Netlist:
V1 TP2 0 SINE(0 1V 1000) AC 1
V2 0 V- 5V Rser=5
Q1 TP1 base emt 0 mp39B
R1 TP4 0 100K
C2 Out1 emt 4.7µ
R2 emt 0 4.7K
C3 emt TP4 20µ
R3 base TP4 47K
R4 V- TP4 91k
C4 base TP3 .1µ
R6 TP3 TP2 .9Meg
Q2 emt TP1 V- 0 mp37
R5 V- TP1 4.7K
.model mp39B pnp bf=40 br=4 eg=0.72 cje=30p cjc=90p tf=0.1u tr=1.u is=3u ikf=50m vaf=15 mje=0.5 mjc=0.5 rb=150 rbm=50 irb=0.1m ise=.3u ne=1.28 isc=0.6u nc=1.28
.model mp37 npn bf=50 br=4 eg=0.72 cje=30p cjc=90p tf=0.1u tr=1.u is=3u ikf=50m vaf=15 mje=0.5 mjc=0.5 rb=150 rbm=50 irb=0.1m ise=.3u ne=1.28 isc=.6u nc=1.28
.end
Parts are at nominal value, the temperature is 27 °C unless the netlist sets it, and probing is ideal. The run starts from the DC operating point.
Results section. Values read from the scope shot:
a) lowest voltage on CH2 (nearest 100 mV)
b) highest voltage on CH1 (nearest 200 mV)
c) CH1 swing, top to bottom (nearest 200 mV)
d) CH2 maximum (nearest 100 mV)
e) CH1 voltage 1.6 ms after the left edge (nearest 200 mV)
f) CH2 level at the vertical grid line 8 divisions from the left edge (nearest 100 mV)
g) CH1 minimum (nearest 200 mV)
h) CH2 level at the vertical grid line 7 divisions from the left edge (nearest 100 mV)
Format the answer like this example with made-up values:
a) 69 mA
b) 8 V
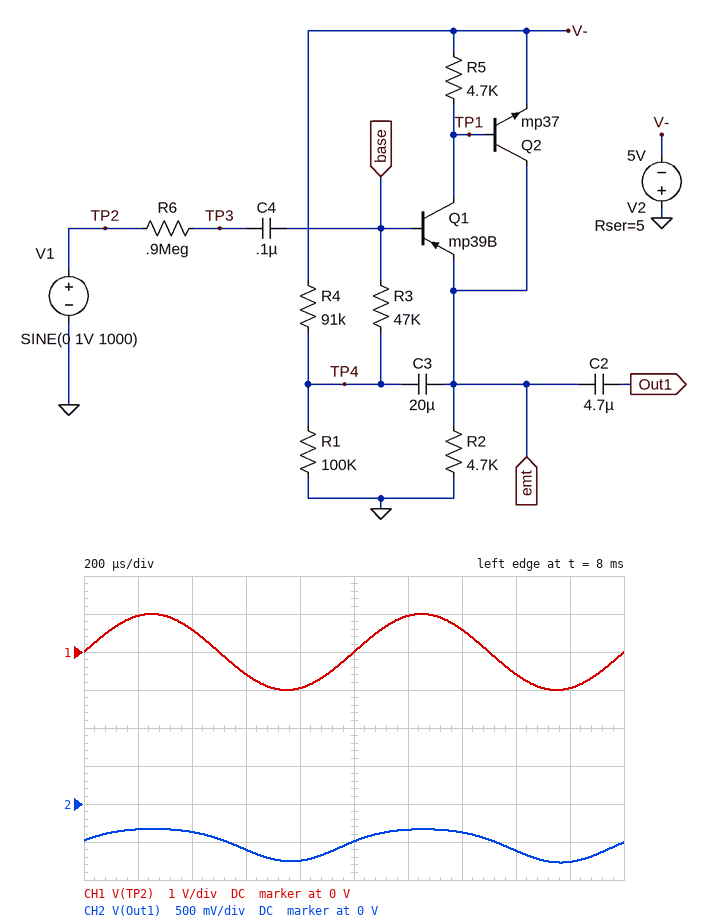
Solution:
a) -800 mV
b) 1.0 V
c) 2.0 V
d) -300 mV
e) -600 mV
f) -600 mV
g) -1.0 V
h) -400 mV
